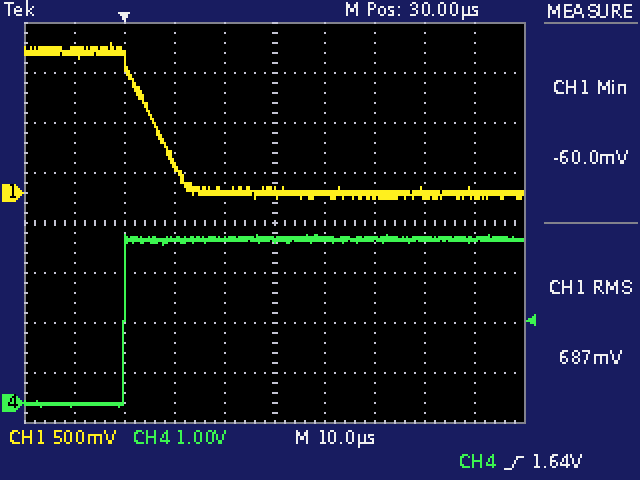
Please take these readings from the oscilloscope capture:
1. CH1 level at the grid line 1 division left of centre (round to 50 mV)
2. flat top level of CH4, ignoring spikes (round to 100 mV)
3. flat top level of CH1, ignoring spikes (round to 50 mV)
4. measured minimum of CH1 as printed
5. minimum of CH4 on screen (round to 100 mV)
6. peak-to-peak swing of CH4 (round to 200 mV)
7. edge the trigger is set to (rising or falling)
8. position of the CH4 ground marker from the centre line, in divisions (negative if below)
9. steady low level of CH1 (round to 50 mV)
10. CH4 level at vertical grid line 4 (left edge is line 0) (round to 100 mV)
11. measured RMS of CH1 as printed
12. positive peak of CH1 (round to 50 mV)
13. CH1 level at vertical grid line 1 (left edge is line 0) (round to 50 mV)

0 mV
3.3 V
1.40 V
-60.0 mV
-100 mV
3.4 V
rising
-3.6 div
0 mV
3.3 V
687 mV
1.50 V
1.40 V
